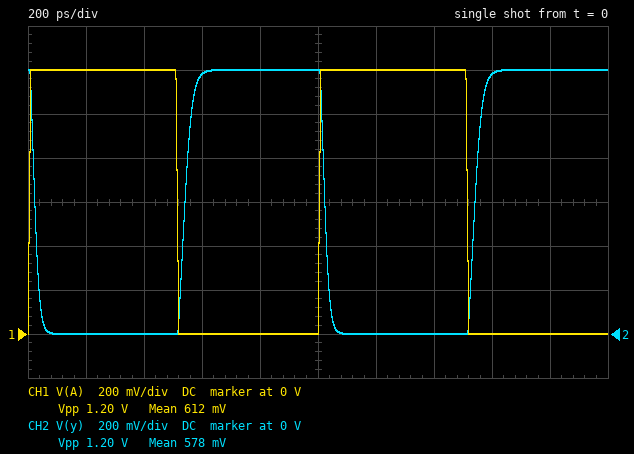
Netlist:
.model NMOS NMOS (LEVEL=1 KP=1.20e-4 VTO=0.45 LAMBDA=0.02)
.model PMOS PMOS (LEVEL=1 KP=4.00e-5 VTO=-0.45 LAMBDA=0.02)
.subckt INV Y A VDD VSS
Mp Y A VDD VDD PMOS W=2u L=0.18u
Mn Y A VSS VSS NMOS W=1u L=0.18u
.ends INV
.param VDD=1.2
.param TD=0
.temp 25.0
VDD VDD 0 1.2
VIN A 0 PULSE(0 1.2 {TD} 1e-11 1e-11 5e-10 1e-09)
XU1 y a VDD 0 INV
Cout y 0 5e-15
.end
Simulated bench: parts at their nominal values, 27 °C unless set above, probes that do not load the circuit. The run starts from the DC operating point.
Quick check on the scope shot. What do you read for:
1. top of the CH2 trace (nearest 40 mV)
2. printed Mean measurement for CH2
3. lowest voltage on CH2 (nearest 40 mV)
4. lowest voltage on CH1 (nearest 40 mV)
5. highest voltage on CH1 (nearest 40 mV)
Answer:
1.20 V
578 mV
0 V
0 V
1.20 V
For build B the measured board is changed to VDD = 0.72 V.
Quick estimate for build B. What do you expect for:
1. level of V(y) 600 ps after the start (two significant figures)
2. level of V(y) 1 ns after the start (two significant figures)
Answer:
260 mV
720 mV
